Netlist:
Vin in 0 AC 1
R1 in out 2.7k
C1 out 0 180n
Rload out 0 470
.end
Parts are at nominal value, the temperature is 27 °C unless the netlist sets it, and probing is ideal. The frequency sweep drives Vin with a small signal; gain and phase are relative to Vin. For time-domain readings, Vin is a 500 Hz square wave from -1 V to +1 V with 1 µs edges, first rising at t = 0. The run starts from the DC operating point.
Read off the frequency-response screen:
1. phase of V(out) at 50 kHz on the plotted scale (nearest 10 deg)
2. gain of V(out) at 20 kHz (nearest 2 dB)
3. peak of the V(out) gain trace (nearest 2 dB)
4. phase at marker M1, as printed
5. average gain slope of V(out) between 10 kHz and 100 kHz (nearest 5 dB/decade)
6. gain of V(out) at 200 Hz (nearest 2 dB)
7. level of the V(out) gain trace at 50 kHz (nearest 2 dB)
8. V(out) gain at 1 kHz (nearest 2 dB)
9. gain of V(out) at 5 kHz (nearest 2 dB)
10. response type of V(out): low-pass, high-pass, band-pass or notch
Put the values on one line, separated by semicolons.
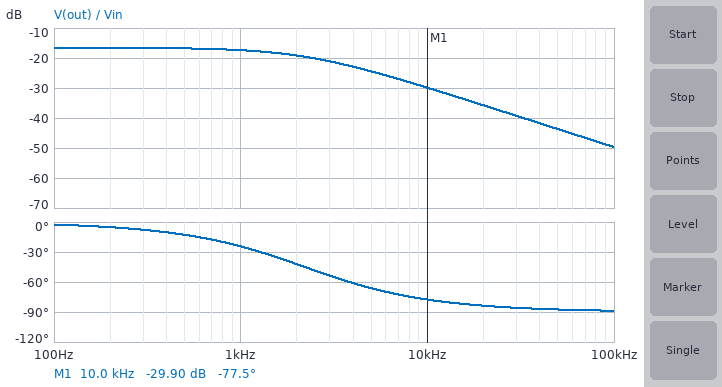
-90 deg; -36 dB; -16 dB; -77.5 deg; -20 dB/decade; -16 dB; -44 dB; -18 dB; -24 dB; low-pass
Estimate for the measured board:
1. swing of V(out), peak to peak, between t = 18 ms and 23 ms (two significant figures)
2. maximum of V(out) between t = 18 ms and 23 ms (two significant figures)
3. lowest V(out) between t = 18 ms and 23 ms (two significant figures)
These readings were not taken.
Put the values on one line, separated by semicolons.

300 mV; 150 mV; -150 mV
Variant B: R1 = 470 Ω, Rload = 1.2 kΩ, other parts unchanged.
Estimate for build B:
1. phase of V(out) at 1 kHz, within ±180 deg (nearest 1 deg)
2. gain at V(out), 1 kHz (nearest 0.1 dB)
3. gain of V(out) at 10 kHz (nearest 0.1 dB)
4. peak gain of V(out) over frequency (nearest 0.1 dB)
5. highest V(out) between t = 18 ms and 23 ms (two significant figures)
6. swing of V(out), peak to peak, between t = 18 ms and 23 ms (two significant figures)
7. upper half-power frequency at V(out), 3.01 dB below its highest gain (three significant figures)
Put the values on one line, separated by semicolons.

-21 deg; -3.5 dB; -14.8 dB; -2.9 dB; 720 mV; 1.4 V; 2.62 kHz
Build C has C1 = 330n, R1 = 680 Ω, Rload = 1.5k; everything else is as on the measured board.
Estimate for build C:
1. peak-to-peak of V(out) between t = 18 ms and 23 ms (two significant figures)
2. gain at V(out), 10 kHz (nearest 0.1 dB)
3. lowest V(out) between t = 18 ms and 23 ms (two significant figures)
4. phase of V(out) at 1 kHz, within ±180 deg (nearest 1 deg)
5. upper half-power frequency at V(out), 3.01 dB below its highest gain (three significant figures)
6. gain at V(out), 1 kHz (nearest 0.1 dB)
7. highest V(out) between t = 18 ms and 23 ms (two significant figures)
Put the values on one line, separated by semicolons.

1.4 V; -23.0 dB; -690 mV; -44 deg; 1.03 kHz; -6.1 dB; 690 mV
